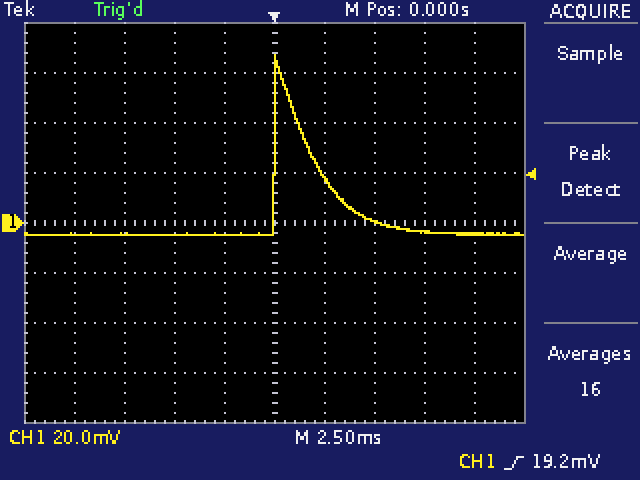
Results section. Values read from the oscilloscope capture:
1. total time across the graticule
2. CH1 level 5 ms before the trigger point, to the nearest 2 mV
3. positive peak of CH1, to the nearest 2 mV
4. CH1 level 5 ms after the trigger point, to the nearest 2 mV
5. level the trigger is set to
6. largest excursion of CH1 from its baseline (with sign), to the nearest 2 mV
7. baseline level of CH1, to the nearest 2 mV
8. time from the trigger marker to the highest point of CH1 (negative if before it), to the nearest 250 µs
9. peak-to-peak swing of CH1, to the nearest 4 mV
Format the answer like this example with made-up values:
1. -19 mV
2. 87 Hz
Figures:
1. 25 ms
2. -4 mV
3. 68 mV
4. 0 mV
5. 19.2 mV
6. +72 mV
7. -4 mV
8. 0.00 ms
9. 72 mV
